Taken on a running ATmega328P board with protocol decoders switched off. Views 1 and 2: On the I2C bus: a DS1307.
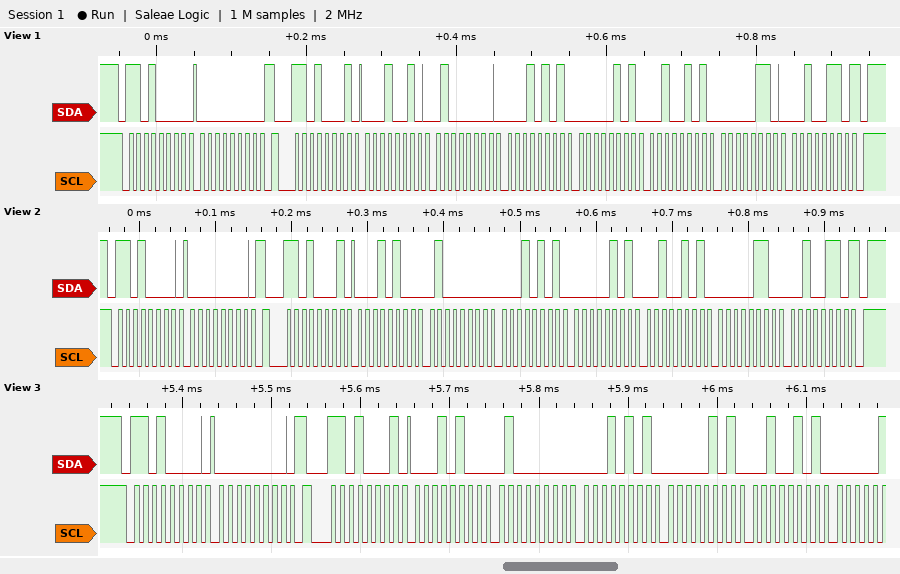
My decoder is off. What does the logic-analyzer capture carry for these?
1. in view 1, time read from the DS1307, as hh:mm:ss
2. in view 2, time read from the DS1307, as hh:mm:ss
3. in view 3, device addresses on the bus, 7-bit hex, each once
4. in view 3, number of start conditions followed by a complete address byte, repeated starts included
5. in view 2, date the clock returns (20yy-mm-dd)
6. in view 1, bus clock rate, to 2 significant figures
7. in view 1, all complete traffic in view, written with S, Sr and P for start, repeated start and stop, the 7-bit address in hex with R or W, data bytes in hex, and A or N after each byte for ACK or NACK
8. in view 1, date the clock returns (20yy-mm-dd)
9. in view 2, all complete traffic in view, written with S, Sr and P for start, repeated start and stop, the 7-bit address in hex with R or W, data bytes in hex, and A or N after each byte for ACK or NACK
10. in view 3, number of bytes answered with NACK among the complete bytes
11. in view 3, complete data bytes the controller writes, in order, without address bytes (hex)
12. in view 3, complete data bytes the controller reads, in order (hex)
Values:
15:40:12
15:40:14
0x68
2
2026-06-25
100 kHz
S 68W A 00 A Sr 68R A 12 A 40 A 15 A 05 A 25 A 06 A 26 N P
2026-06-25
S 68W A 00 A Sr 68R A 14 A 40 A 15 A 05 A 25 A 06 A 26 N P
0
00
14 40 15 05 25
